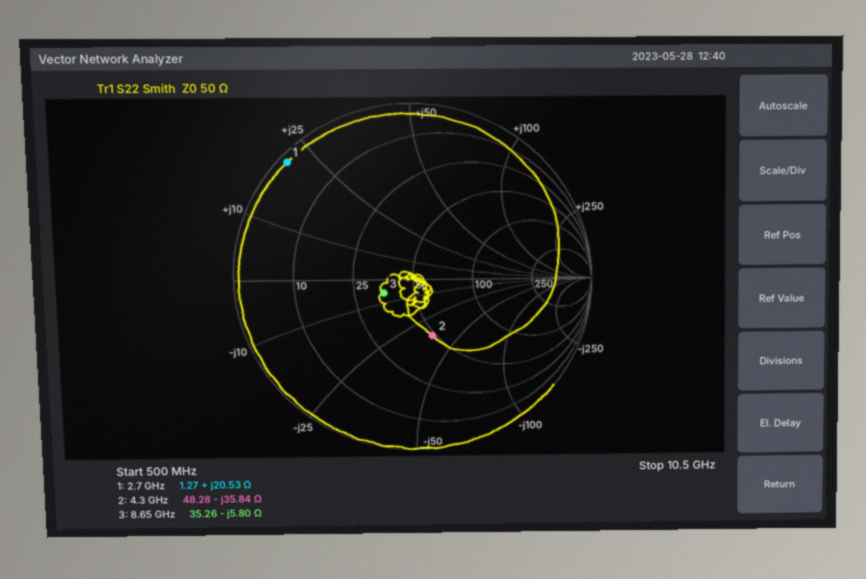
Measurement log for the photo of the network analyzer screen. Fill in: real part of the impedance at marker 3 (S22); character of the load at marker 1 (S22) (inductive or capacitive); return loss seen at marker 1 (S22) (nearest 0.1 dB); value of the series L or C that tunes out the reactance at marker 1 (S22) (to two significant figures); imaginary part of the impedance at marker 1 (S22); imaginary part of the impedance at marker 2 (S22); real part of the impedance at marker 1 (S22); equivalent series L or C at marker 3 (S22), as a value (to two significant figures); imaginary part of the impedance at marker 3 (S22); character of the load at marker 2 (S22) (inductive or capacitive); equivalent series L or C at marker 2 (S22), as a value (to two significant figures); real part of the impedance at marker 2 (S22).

35.26 Ω
inductive
0.4 dB
2.9 pF
+20.53 Ω
-35.84 Ω
1.27 Ω
3.2 pF
-5.80 Ω
capacitive
1.0 pF
48.28 Ω
